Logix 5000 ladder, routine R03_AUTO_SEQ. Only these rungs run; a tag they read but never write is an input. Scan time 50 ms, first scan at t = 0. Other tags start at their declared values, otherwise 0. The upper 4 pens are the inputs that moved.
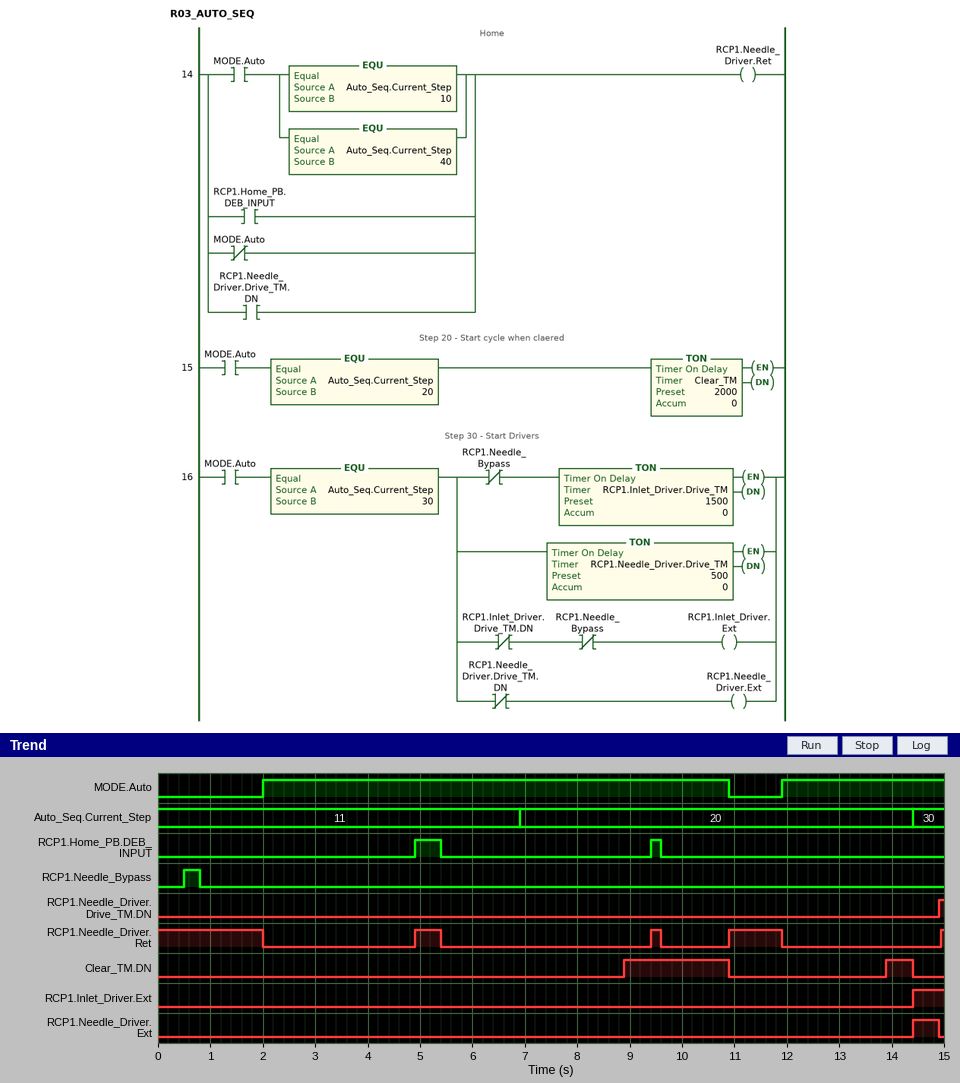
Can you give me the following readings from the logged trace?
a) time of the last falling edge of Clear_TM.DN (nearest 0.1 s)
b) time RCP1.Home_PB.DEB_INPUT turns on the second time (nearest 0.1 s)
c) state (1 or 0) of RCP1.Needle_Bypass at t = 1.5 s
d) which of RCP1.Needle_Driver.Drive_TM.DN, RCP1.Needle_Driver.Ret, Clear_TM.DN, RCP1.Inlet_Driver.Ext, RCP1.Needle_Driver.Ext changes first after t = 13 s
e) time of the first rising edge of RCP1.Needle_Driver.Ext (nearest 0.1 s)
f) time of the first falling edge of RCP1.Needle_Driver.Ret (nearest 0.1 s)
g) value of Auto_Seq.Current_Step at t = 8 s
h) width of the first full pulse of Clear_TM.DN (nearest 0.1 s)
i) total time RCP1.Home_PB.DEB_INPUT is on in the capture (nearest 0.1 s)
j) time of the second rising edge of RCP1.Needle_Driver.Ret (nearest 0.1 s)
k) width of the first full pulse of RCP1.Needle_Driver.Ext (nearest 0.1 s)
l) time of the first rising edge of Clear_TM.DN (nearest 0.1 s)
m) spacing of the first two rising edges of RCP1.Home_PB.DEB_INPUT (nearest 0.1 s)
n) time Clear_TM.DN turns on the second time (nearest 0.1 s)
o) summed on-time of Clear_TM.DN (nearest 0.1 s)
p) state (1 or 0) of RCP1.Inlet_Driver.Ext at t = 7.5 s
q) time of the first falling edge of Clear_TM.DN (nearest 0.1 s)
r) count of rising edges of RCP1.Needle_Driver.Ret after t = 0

14.4 s
9.4 s
0
Clear_TM.DN
14.4 s
2.0 s
20
2.0 s
0.7 s
9.4 s
0.5 s
8.9 s
4.5 s
13.9 s
2.5 s
0
10.9 s
4
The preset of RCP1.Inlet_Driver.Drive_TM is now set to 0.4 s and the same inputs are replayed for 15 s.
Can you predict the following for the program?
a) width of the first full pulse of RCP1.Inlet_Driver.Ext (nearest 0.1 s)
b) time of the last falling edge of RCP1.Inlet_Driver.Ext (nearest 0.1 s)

0.4 s
14.8 s
